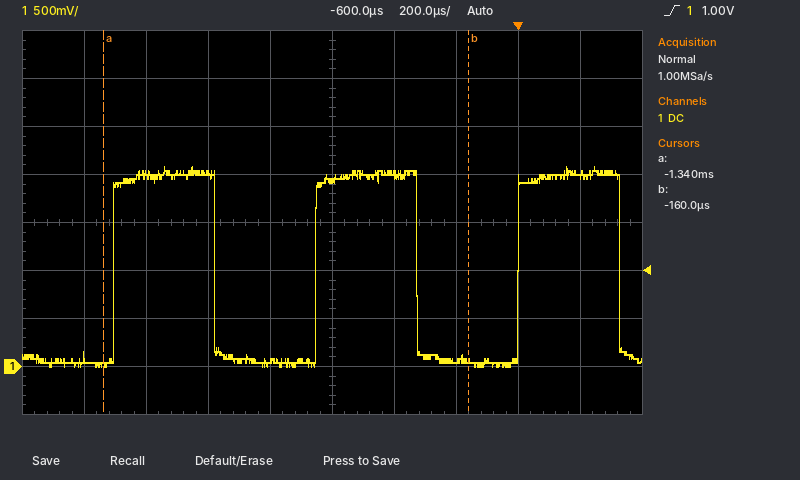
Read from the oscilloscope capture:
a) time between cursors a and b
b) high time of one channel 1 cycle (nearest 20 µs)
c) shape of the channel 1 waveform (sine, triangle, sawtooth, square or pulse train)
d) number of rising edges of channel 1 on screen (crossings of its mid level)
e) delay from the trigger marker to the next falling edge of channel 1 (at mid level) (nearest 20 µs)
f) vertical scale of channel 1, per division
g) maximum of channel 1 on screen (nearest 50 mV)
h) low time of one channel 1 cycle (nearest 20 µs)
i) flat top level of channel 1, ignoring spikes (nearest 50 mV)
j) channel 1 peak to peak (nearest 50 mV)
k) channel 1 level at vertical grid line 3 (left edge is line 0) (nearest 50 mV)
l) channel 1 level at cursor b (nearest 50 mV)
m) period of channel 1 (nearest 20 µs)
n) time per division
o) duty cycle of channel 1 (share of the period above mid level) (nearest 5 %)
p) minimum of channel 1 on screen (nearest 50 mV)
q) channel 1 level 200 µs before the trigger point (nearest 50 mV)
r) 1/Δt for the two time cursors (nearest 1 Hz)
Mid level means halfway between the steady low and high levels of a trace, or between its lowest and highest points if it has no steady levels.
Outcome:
1.18 ms
320 µs
square
3
320 µs
500 mV
2.10 V
320 µs
2.00 V
2.10 V
2.00 V
50 mV
660 µs
200 µs
50 %
0 mV
50 mV
847 Hz
